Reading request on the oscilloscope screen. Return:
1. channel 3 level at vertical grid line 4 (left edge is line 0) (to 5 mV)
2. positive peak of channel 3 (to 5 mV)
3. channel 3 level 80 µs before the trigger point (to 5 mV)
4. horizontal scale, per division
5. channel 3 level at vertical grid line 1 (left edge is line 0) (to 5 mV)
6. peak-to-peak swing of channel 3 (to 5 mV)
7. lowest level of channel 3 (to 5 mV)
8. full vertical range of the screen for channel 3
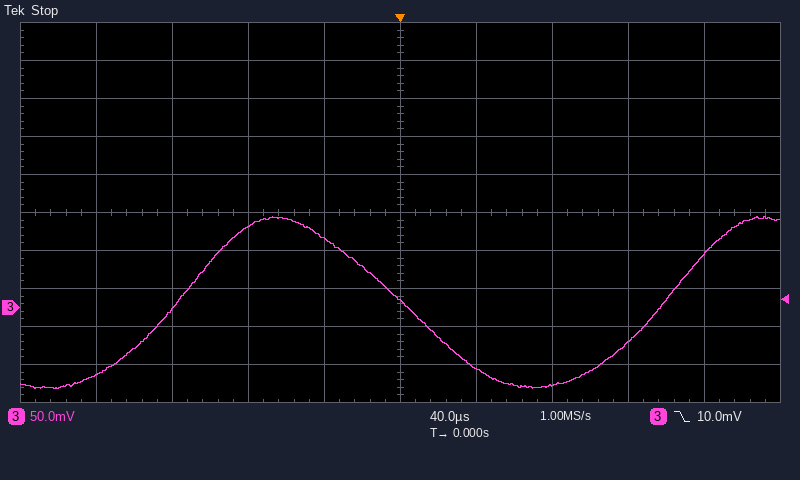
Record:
90 mV
120 mV
105 mV
40 µs
-90 mV
225 mV
-105 mV
500 mV
